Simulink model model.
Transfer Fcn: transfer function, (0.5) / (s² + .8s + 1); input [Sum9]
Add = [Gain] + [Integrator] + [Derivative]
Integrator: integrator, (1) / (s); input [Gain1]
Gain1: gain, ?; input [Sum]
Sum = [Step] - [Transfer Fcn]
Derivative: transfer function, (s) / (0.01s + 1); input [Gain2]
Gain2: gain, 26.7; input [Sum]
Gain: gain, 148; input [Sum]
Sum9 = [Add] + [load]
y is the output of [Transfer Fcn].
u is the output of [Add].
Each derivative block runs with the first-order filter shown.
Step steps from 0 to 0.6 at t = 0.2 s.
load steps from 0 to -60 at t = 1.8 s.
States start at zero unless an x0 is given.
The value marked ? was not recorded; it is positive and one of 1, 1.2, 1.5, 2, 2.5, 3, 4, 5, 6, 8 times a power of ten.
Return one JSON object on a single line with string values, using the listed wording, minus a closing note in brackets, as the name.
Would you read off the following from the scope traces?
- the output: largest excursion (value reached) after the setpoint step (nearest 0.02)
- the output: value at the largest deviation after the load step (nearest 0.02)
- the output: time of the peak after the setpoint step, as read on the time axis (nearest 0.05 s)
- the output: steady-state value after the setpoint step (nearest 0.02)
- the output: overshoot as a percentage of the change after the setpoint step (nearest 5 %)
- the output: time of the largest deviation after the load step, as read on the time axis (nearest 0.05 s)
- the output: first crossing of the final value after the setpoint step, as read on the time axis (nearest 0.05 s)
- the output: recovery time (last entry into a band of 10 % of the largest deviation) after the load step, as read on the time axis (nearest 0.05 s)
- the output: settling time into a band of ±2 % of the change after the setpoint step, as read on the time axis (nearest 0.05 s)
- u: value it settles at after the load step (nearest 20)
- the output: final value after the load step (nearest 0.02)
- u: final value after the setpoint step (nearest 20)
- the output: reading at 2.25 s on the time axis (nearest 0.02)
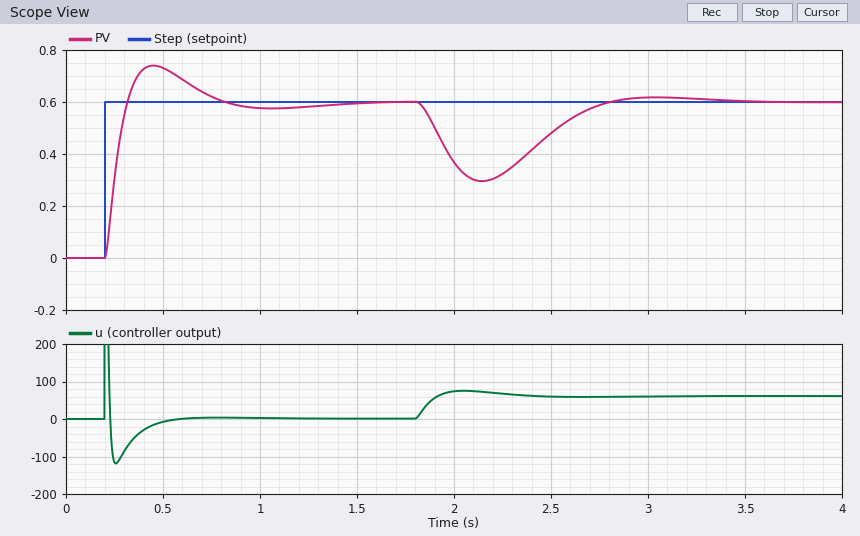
{"the output: largest excursion (value reached) after the setpoint step": "0.74", "the output: value at the largest deviation after the load step": "0.30", "the output: time of the peak after the setpoint step, as read on the time axis": "0.45 s", "the output: steady-state value after the setpoint step": "0.60", "the output: overshoot as a percentage of the change after the setpoint step": "25 %", "the output: time of the largest deviation after the load step, as read on the time axis": "2.15 s", "the output: first crossing of the final value after the setpoint step, as read on the time axis": "0.30 s", "the output: recovery time (last entry into a band of 10 % of the largest deviation) after the load step, as read on the time axis": "2.70 s", "the output: settling time into a band of ±2 % of the change after the setpoint step, as read on the time axis": "1.35 s", "u: value it settles at after the load step": "60", "the output: final value after the load step": "0.60", "u: final value after the setpoint step": "0", "the output: reading at 2.25 s on the time axis": "0.32"}
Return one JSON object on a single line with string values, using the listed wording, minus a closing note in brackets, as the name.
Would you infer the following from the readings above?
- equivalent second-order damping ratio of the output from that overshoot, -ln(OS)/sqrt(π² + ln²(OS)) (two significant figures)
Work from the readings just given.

{"equivalent second-order damping ratio of the output from that overshoot, -ln(OS)/sqrt(π² + ln²(OS))": "0.40"}
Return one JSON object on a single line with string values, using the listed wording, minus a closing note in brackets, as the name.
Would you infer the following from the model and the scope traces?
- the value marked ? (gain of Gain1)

{"the value marked ?": "400"}
